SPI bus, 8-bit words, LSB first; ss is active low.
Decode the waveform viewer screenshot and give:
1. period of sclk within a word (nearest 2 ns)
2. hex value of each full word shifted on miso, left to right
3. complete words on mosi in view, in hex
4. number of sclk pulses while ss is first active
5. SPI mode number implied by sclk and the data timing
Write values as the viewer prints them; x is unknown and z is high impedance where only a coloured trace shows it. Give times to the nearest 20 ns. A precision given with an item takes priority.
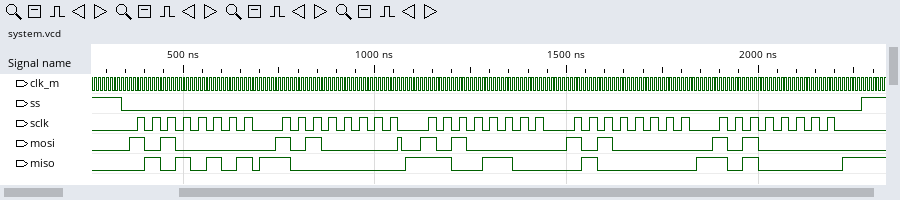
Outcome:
40 ns
AA, 01, 33, 02, 05
05, 05, 05, 05, 05
40
0
